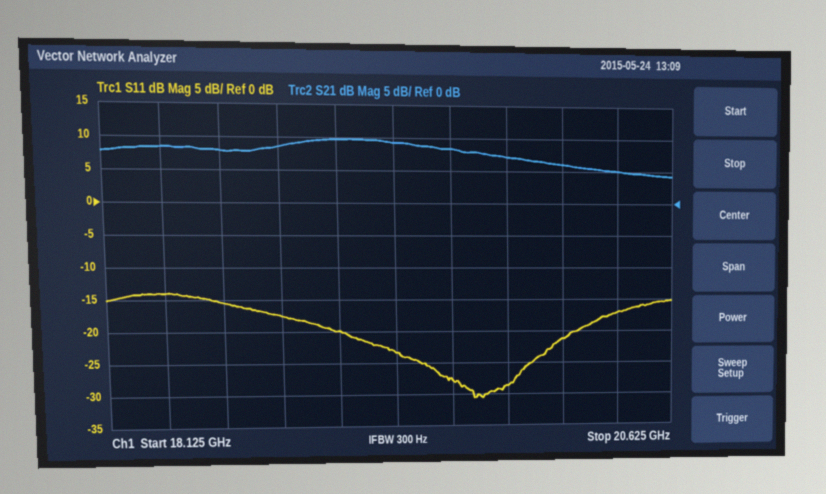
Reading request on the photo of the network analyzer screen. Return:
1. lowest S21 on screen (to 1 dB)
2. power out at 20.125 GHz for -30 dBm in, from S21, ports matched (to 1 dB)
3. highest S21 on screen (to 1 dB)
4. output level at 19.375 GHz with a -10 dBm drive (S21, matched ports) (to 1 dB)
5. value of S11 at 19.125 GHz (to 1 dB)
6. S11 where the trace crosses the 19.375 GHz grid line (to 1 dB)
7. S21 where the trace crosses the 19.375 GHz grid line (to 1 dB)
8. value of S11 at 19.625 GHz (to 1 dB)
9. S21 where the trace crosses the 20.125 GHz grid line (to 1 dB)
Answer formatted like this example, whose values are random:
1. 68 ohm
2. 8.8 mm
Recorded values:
1. 4 dB
2. -24 dBm
3. 10 dB
4. -1 dBm
5. -20 dB
6. -23 dB
7. 9 dB
8. -28 dB
9. 6 dB
